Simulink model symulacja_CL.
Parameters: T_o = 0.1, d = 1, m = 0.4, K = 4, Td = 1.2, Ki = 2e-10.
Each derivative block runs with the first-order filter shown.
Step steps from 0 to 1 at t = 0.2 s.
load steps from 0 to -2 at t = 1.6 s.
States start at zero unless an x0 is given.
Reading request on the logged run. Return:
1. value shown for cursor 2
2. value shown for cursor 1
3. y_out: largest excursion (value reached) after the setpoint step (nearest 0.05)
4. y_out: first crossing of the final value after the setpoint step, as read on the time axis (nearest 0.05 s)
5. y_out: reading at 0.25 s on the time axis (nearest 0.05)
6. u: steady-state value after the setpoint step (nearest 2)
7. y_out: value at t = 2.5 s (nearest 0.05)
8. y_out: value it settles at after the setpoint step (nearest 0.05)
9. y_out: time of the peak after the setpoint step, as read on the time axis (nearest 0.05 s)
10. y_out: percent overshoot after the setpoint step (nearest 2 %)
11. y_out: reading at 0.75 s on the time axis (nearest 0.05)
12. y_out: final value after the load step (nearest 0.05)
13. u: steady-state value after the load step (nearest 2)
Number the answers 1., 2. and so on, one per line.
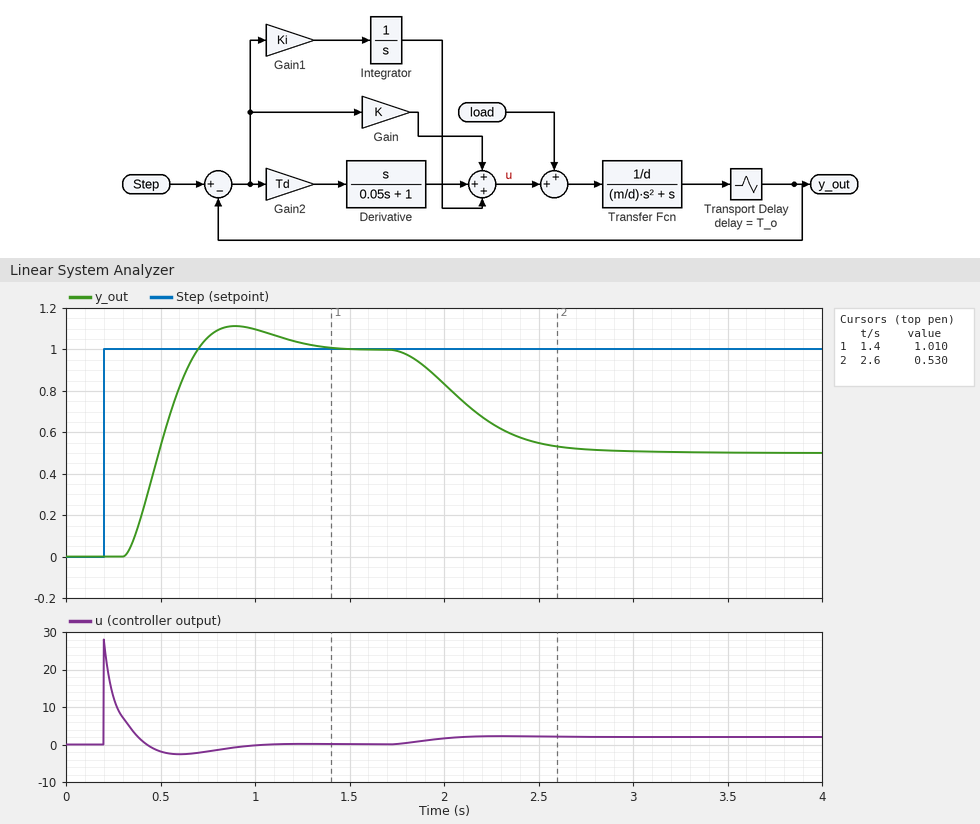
1. 0.530
2. 1.010
3. 1.10
4. 0.70 s
5. 0.00
6. 0
7. 0.55
8. 1.00
9. 0.90 s
10. 12 %
11. 1.05
12. 0.50
13. 2
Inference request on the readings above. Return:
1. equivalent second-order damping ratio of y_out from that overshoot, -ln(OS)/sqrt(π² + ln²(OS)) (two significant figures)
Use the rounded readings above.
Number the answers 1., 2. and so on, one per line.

1. 0.56
